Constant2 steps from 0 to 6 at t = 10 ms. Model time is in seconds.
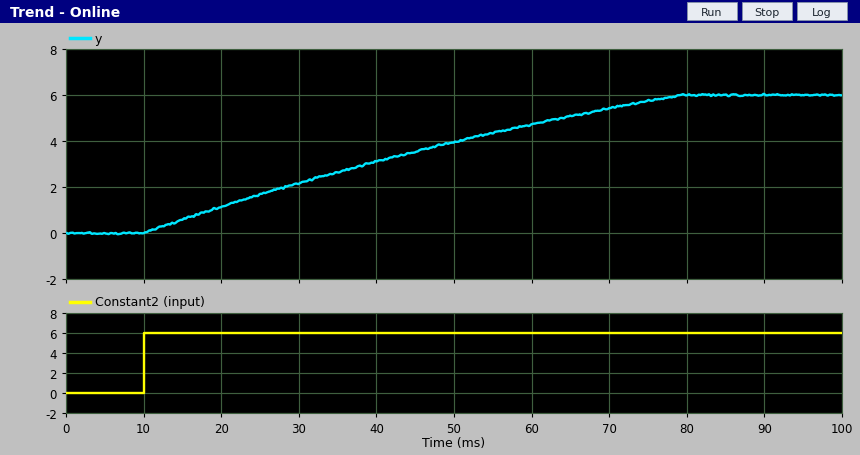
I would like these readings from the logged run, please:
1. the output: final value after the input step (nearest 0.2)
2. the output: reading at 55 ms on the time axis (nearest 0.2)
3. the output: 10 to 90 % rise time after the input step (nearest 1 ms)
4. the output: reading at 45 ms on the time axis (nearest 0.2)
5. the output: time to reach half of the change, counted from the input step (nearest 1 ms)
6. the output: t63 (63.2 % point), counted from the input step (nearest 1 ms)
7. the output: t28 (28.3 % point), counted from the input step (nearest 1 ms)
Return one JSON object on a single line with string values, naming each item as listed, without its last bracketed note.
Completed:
{"the output: final value after the input step": "6.0", "the output: reading at 55 ms on the time axis": "4.4", "the output: 10 to 90 % rise time after the input step": "55 ms", "the output: reading at 45 ms on the time axis": "3.6", "the output: time to reach half of the change, counted from the input step": "29 ms", "the output: t63 (63.2 % point), counted from the input step": "38 ms", "the output: t28 (28.3 % point), counted from the input step": "15 ms"}
